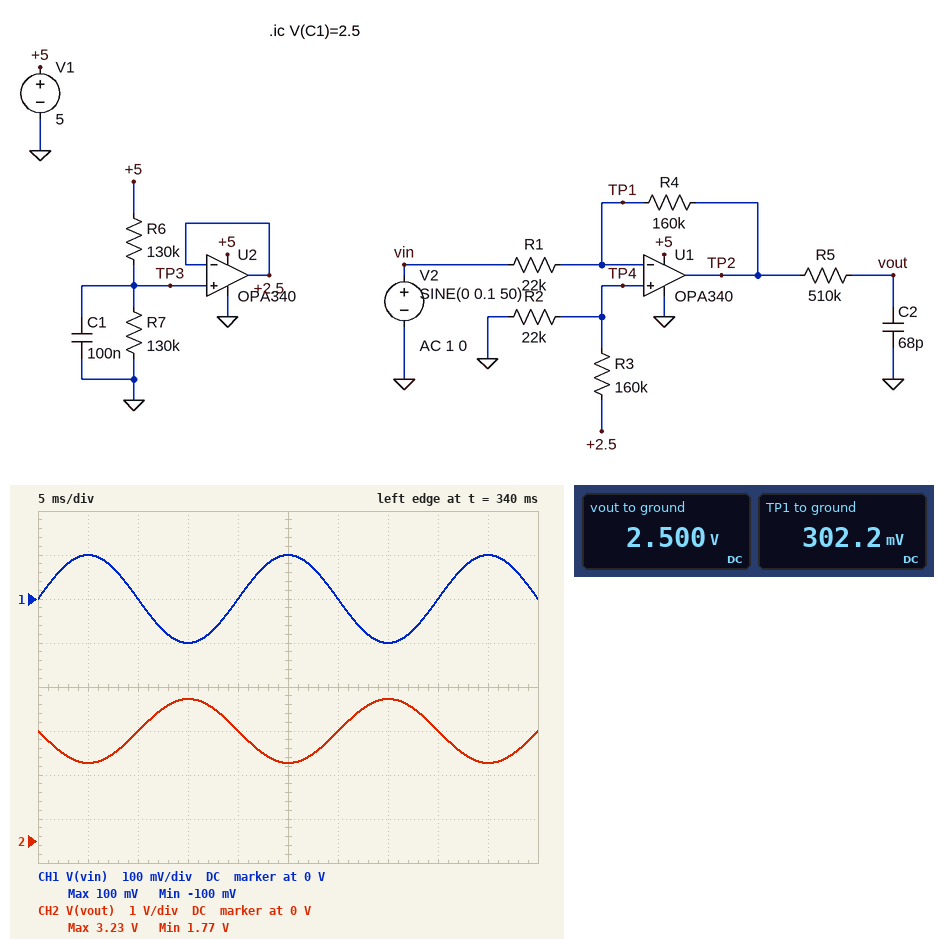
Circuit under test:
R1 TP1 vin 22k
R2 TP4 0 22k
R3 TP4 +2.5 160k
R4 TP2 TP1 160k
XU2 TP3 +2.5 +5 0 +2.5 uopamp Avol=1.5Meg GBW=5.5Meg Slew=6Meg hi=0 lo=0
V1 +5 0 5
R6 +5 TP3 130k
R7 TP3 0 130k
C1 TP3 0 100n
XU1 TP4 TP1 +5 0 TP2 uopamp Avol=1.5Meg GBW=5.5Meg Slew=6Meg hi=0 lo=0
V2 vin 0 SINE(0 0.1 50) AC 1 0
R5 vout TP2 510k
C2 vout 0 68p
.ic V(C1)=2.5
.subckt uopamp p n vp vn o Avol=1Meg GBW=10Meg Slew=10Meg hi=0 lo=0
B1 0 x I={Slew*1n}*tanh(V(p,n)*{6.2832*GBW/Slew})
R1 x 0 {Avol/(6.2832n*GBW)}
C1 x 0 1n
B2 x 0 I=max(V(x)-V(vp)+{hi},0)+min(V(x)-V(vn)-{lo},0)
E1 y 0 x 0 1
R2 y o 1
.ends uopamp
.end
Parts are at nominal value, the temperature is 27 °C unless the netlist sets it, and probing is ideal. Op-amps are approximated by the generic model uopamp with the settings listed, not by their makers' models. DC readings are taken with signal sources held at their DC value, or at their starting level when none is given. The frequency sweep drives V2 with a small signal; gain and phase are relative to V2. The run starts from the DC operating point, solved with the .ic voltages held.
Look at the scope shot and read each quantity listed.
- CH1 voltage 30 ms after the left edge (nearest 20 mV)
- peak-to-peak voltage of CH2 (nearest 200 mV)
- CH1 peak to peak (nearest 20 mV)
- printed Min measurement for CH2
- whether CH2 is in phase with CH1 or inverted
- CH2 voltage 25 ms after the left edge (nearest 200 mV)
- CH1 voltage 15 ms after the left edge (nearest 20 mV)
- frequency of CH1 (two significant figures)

0 V
1.4 V
200 mV
1.77 V
inverted
1.8 V
-100 mV
50 Hz
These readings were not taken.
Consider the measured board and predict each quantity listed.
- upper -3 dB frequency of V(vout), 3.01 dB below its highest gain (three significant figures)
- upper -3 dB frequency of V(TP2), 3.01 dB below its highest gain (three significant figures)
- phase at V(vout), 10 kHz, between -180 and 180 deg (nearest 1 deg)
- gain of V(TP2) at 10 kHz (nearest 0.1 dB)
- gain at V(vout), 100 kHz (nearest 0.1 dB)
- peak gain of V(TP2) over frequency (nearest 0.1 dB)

4.59 kHz
665 kHz
114 deg
17.2 dB
-9.6 dB
17.2 dB
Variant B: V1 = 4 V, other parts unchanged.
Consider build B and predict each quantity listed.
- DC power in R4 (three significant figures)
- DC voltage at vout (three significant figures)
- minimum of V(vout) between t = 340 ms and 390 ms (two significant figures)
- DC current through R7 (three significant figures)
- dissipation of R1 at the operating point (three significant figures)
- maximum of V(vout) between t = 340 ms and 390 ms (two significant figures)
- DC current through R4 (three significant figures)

19.3 µW
2.00 V
1.3 V
15.4 µA
2.66 µW
2.7 V
11.0 µA
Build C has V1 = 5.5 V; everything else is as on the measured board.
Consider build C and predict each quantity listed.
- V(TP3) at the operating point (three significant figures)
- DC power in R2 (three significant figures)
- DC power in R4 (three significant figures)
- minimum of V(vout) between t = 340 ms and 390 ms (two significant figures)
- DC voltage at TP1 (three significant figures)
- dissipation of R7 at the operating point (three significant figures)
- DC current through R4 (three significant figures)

2.75 V
5.02 µW
36.5 µW
2.0 V
332 mV
58.2 µW
15.1 µA
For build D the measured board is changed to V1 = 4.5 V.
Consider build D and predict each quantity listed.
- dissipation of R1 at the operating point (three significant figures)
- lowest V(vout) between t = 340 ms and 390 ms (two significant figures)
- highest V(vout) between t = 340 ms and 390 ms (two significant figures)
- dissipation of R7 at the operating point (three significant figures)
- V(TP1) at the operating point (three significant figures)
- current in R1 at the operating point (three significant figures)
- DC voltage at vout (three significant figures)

3.36 µW
1.5 V
3.0 V
38.9 µW
272 mV
12.4 µA
2.25 V
